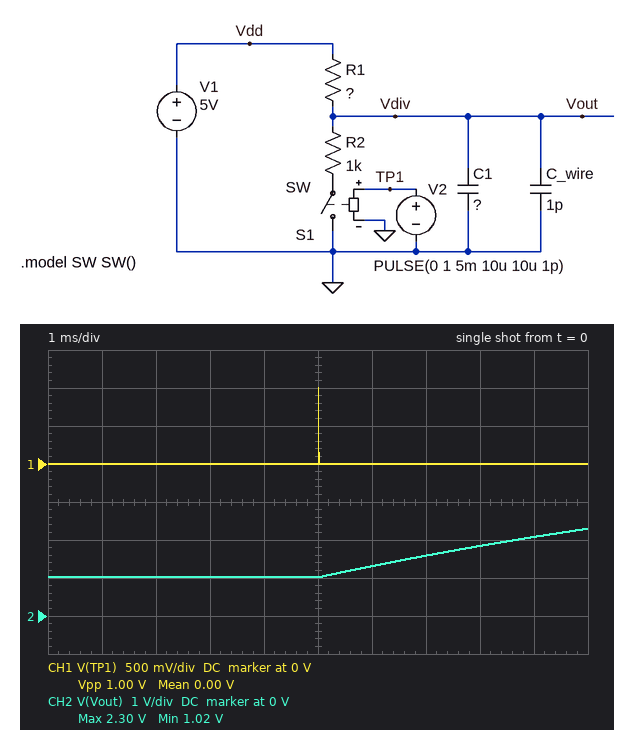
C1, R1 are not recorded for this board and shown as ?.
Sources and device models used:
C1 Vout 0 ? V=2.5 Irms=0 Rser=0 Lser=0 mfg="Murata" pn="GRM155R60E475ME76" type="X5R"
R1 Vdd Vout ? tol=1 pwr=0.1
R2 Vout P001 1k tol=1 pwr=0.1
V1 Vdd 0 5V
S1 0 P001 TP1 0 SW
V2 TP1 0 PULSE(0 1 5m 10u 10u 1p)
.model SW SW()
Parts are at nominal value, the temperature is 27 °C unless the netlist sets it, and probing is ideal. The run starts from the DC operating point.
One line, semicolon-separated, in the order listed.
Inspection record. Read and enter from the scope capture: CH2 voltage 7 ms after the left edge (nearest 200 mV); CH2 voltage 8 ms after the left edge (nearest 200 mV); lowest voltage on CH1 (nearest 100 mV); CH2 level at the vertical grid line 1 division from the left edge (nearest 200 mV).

1.6 V; 1.8 V; 0 V; 1.0 V
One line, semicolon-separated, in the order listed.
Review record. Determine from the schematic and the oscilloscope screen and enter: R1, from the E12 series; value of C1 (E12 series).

3.9 kΩ; 3.3 µF
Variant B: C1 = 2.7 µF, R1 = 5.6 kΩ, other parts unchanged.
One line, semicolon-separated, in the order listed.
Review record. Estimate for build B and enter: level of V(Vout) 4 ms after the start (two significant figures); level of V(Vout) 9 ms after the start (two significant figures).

760 mV; 1.7 V
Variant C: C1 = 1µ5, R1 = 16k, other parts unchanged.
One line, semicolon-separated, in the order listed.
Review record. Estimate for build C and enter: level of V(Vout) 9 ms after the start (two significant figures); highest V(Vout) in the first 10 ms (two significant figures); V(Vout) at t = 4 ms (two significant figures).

1.0 V; 1.2 V; 290 mV
